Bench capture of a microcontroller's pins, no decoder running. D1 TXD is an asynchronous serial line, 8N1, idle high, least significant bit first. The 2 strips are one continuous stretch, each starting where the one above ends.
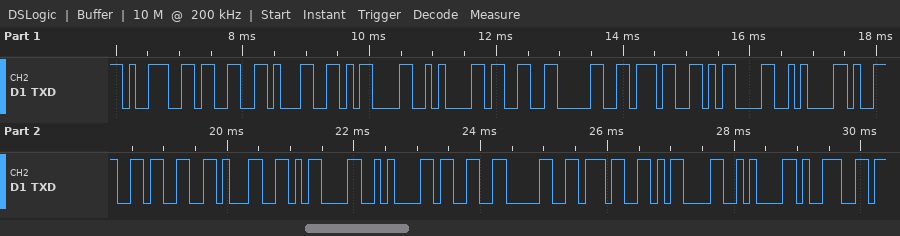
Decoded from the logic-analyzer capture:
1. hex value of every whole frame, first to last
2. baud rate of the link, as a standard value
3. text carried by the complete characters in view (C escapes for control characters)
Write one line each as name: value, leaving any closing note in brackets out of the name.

hex value of every whole frame, first to last: 39 33 31 0D 0A 33 30 37 0D 0A 39 33 31 0D 0A 33 30 37 0D 0A 39
baud rate of the link, as a standard value: 9600 baud
text carried by the complete characters in view: "931\r\n307\r\n931\r\n307\r\n9"
